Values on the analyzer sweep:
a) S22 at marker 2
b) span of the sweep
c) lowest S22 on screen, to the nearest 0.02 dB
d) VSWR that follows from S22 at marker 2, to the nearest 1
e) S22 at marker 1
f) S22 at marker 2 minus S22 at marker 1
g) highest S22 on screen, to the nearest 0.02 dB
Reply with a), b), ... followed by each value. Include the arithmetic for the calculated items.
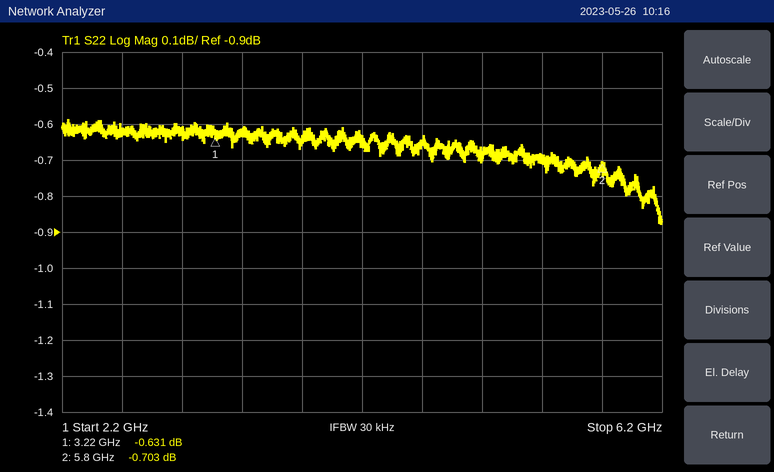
a) -0.703 dB
b) 4 GHz
c) -0.88 dB
d) (1 + 0.9223)/(1 − 0.9223) ≈ 25
e) -0.631 dB
f) -0.703 − (-0.631) = -0.072 dB
g) -0.58 dB
